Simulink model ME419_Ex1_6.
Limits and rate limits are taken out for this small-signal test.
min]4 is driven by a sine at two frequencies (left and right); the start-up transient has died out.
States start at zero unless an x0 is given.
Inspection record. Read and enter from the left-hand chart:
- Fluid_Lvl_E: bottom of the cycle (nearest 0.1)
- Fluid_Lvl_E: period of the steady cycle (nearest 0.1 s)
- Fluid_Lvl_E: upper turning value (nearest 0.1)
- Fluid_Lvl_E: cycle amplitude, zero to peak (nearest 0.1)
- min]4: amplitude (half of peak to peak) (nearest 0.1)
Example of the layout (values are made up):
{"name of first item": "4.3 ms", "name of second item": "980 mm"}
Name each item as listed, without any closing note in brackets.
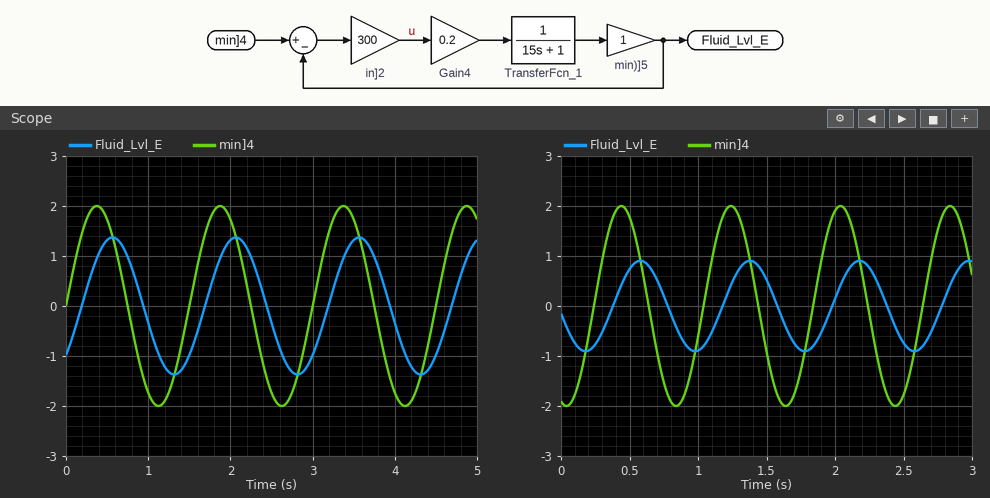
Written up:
{"Fluid_Lvl_E: bottom of the cycle": "-1.4", "Fluid_Lvl_E: period of the steady cycle": "1.5 s", "Fluid_Lvl_E: upper turning value": "1.4", "Fluid_Lvl_E: cycle amplitude, zero to peak": "1.4", "min]4: amplitude (half of peak to peak)": "2.0"}
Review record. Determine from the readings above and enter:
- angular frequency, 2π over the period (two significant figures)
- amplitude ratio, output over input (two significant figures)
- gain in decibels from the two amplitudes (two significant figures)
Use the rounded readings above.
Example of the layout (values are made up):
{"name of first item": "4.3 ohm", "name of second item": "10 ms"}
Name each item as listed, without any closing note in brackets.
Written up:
{"angular frequency, 2π over the period": "4.2 rad/s", "amplitude ratio, output over input": "0.70", "gain in decibels from the two amplitudes": "-3.1 dB"}
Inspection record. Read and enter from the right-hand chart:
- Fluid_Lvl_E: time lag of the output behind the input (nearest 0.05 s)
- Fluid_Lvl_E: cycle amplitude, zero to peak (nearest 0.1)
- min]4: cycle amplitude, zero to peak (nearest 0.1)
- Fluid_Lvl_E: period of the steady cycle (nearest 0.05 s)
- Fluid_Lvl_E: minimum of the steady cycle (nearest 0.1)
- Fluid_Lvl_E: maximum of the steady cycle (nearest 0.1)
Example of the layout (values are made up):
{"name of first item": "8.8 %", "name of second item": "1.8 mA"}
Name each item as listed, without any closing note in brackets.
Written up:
{"Fluid_Lvl_E: time lag of the output behind the input": "0.15 s", "Fluid_Lvl_E: cycle amplitude, zero to peak": "0.9", "min]4: cycle amplitude, zero to peak": "2.0", "Fluid_Lvl_E: period of the steady cycle": "0.80 s", "Fluid_Lvl_E: minimum of the steady cycle": "-0.9", "Fluid_Lvl_E: maximum of the steady cycle": "0.9"}
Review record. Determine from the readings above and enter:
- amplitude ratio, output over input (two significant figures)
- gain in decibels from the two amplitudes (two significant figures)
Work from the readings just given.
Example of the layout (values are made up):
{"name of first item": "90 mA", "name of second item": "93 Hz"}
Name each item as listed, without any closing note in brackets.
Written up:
{"amplitude ratio, output over input": "0.45", "gain in decibels from the two amplitudes": "-6.9 dB"}
